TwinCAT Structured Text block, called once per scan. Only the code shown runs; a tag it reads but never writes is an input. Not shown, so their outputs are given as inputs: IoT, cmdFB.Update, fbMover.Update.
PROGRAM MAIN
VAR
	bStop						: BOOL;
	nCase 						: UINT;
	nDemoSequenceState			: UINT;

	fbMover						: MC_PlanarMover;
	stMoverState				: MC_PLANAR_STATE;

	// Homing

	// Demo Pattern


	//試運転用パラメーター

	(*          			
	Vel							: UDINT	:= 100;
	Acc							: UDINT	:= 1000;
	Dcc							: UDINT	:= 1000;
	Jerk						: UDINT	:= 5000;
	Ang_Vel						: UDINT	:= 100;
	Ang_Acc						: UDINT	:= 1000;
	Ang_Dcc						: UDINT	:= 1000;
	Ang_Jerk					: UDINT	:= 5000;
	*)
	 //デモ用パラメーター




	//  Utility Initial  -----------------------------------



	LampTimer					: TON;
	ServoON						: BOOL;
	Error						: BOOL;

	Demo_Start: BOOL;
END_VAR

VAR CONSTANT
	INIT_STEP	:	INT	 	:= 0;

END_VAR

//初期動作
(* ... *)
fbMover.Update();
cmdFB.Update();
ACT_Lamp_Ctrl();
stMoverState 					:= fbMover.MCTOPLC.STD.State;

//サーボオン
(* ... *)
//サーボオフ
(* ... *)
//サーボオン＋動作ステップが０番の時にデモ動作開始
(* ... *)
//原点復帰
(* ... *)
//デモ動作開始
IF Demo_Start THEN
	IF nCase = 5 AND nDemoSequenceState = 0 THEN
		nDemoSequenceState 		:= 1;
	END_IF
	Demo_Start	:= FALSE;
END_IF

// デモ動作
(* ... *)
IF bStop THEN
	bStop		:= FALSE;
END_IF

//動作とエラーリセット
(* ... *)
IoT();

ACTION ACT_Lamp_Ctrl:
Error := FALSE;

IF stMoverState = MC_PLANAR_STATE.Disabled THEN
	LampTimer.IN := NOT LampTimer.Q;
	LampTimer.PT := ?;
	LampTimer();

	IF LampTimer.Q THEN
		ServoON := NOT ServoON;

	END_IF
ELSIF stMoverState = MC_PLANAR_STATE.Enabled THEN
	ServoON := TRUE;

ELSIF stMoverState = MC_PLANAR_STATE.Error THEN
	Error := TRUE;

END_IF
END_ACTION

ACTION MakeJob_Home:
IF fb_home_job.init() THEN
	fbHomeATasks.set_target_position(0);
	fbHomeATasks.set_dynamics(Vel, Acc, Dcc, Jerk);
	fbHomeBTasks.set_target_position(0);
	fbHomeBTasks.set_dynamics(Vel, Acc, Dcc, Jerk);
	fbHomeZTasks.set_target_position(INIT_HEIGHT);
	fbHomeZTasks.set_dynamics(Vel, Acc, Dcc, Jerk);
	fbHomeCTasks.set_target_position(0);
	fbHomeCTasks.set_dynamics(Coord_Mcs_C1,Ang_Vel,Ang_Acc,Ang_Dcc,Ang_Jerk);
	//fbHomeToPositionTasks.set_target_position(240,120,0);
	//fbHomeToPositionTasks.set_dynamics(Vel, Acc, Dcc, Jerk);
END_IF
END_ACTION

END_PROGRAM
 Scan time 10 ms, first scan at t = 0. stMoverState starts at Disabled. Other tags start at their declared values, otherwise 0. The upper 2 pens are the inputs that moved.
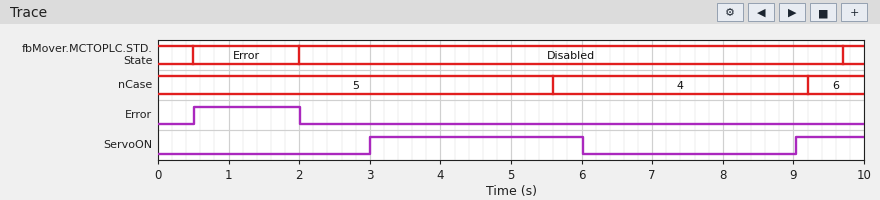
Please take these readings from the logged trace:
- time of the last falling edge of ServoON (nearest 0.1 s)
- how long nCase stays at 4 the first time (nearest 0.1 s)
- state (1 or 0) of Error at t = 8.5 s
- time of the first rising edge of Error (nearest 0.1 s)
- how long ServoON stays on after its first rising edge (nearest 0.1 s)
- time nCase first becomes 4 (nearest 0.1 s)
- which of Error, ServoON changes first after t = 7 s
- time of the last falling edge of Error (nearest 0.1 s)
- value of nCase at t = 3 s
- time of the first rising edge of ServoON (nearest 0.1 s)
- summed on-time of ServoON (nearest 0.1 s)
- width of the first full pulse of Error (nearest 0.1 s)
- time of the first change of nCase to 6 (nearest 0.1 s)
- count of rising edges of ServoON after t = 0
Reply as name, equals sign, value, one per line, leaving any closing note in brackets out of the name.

time of the last falling edge of ServoON = 6.0 s
how long nCase stays at 4 the first time = 3.6 s
state (1 or 0) of Error at t = 8.5 s = 0
time of the first rising edge of Error = 0.5 s
how long ServoON stays on after its first rising edge = 3.0 s
time nCase first becomes 4 = 5.6 s
which of Error, ServoON changes first after t = 7 s = ServoON
time of the last falling edge of Error = 2.0 s
value of nCase at t = 3 s = 5
time of the first rising edge of ServoON = 3.0 s
summed on-time of ServoON = 4.0 s
width of the first full pulse of Error = 1.5 s
time of the first change of nCase to 6 = 9.2 s
count of rising edges of ServoON after t = 0 = 2
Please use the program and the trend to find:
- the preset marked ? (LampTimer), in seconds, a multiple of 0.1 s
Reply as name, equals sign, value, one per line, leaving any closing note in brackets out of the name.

the preset marked ? (LampTimer), in seconds, a multiple of 0.1 s = 3.0 s
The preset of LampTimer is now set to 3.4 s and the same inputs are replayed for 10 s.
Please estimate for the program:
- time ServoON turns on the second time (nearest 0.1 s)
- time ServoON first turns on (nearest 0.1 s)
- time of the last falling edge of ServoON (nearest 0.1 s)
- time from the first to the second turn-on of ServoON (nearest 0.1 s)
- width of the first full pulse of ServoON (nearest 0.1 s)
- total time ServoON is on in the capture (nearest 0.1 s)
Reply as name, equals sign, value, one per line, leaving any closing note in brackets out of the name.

time ServoON turns on the second time = 9.7 s
time ServoON first turns on = 3.4 s
time of the last falling edge of ServoON = 6.8 s
time from the first to the second turn-on of ServoON = 6.3 s
width of the first full pulse of ServoON = 3.4 s
total time ServoON is on in the capture = 3.7 s
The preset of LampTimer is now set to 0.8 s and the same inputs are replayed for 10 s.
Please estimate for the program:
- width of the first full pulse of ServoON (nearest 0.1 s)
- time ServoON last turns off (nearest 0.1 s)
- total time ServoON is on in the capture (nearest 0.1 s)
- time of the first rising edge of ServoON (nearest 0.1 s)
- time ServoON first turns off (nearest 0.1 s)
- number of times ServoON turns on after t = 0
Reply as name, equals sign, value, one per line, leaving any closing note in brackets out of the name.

width of the first full pulse of ServoON = 0.8 s
time ServoON last turns off = 9.4 s
total time ServoON is on in the capture = 4.4 s
time of the first rising edge of ServoON = 2.0 s
time ServoON first turns off = 2.8 s
number of times ServoON turns on after t = 0 = 6
